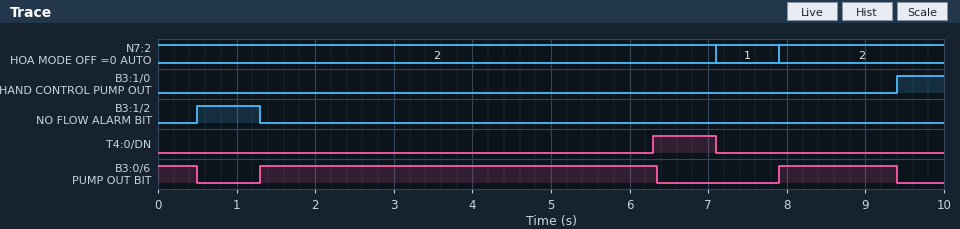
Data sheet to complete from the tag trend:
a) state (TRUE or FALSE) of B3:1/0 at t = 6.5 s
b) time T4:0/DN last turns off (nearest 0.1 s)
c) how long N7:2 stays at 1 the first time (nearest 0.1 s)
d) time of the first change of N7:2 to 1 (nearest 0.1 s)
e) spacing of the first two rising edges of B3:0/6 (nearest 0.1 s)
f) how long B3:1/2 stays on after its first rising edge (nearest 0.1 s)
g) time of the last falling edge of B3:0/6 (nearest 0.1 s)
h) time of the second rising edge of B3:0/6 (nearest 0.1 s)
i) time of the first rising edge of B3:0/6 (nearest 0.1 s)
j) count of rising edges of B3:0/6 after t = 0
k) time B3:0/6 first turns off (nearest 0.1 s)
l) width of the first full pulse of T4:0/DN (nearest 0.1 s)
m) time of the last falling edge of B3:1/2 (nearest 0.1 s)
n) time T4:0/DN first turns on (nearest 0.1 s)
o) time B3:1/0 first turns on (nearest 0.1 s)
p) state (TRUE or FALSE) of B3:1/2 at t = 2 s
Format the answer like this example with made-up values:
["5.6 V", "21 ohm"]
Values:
["FALSE", "7.1 s", "0.8 s", "7.1 s", "6.6 s", "0.8 s", "9.4 s", "7.9 s", "1.3 s", "2", "0.5 s", "0.8 s", "1.3 s", "6.3 s", "9.4 s", "FALSE"]
